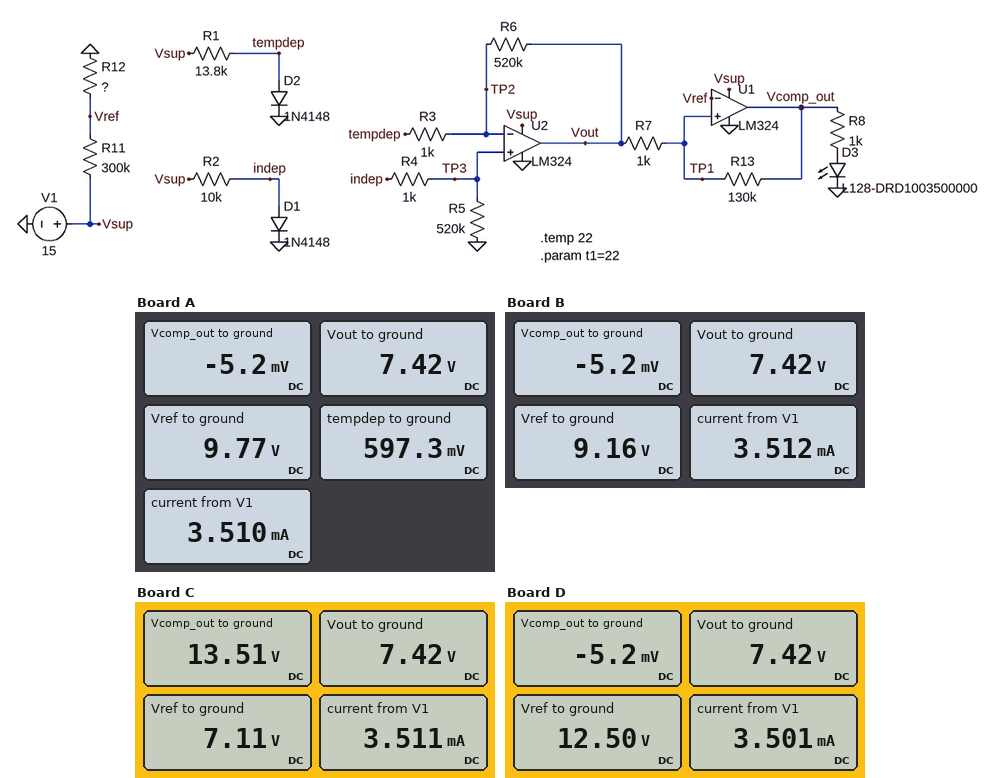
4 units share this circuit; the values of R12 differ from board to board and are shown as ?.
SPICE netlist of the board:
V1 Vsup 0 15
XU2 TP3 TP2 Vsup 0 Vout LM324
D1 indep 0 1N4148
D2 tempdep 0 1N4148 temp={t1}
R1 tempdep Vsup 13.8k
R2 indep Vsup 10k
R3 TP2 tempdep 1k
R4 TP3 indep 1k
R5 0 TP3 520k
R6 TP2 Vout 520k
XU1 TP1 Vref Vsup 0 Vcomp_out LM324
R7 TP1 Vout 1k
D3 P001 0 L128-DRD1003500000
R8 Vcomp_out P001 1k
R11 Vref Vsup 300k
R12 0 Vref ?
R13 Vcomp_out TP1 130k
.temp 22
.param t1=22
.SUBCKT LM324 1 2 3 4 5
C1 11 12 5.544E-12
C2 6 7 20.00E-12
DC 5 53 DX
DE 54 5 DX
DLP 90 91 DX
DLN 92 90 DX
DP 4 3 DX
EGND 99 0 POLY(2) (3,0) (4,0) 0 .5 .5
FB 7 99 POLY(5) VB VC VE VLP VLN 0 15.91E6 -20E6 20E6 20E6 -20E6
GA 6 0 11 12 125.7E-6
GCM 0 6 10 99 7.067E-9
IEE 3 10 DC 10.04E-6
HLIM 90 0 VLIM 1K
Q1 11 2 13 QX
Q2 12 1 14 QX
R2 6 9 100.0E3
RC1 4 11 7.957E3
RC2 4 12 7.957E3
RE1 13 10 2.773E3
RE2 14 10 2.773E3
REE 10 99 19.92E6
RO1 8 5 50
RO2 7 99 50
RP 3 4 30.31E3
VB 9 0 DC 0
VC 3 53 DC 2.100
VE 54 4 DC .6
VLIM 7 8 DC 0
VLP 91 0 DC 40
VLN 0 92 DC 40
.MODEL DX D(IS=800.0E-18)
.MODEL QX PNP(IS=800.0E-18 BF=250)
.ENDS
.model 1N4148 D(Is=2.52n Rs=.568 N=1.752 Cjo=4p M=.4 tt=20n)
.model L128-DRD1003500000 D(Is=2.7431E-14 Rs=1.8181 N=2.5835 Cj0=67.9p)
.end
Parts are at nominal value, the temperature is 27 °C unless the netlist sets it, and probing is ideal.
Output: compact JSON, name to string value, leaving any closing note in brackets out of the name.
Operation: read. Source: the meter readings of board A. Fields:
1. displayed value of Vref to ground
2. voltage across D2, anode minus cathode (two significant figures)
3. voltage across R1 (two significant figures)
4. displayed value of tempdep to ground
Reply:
{"displayed value of Vref to ground": "9.77 V", "voltage across D2, anode minus cathode": "600 mV", "voltage across R1": "14 V", "displayed value of tempdep to ground": "597.3 mV"}
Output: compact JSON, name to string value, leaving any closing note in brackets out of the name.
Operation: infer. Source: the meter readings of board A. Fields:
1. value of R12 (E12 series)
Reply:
{"value of R12": "560 kΩ"}
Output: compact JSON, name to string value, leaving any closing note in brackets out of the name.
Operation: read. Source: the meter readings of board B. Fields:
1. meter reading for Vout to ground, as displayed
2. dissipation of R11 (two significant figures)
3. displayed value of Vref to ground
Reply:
{"meter reading for Vout to ground, as displayed": "7.42 V", "dissipation of R11": "110 µW", "displayed value of Vref to ground": "9.16 V"}
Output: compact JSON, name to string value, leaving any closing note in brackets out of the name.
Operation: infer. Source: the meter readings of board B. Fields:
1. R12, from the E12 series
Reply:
{"R12, from the E12 series": "470 kΩ"}
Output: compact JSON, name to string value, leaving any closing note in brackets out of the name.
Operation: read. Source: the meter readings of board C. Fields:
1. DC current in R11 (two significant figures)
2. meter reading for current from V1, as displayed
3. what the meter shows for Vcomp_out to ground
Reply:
{"DC current in R11": "26 µA", "meter reading for current from V1, as displayed": "3.511 mA", "what the meter shows for Vcomp_out to ground": "13.51 V"}
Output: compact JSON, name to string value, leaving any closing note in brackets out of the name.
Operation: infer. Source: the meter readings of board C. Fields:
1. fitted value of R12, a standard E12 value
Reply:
{"fitted value of R12, a standard E12 value": "270 kΩ"}
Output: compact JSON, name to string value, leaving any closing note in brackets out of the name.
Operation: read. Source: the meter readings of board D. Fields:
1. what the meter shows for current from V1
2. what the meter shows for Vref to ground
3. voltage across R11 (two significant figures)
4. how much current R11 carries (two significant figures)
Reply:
{"what the meter shows for current from V1": "3.501 mA", "what the meter shows for Vref to ground": "12.50 V", "voltage across R11": "2.5 V", "how much current R11 carries": "8.3 µA"}
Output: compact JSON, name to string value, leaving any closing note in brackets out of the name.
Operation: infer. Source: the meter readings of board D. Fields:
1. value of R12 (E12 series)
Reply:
{"value of R12": "1.5 MΩ"}
